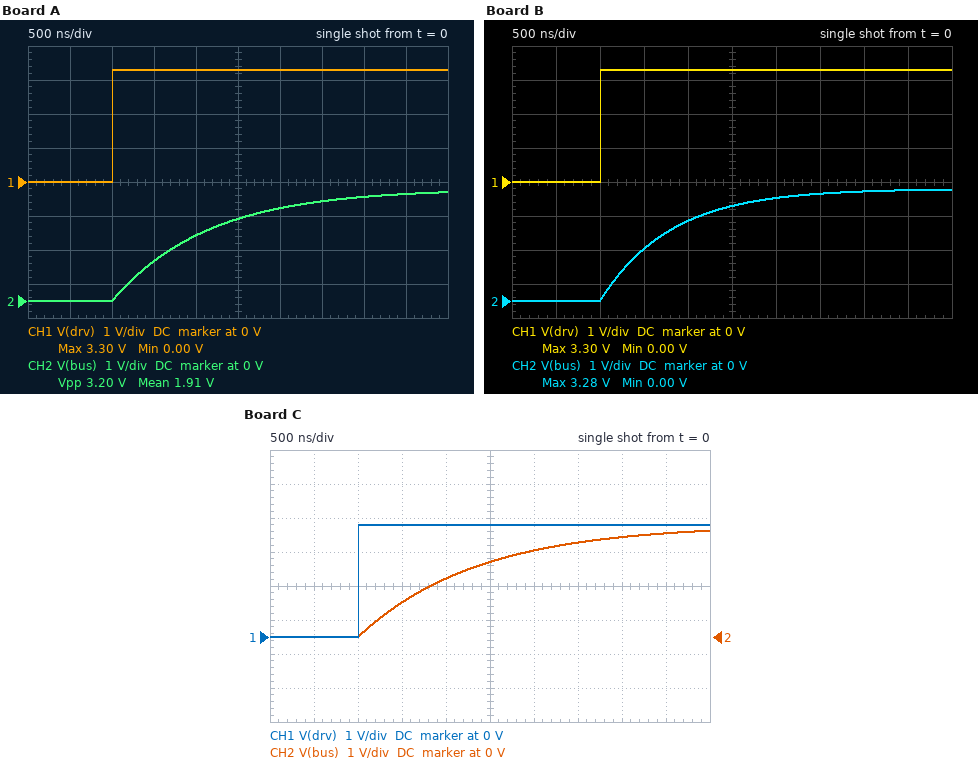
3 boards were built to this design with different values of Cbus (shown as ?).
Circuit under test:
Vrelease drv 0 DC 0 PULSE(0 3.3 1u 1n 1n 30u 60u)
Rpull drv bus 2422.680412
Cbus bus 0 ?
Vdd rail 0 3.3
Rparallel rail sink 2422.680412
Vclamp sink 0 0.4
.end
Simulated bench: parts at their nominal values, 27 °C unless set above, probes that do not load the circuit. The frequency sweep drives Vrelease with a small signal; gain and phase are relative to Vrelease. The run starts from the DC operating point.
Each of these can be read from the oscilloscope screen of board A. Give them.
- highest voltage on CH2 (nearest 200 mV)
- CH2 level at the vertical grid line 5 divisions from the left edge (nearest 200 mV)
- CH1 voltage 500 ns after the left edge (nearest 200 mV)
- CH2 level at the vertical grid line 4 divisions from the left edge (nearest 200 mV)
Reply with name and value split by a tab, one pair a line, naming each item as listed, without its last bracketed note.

highest voltage on CH2	3.2 V
CH2 level at the vertical grid line 5 divisions from the left edge	2.4 V
CH1 voltage 500 ns after the left edge	0 V
CH2 level at the vertical grid line 4 divisions from the left edge	2.0 V
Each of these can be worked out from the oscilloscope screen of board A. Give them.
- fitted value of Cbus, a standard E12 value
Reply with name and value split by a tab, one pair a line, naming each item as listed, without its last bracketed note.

fitted value of Cbus, a standard E12 value	470 pF
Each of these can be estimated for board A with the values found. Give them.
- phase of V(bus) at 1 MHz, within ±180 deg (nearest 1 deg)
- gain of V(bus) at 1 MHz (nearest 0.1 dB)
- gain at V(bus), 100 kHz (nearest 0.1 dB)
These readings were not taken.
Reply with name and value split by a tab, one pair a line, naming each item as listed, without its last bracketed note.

phase of V(bus) at 1 MHz, within ±180 deg	-82 deg
gain of V(bus) at 1 MHz	-17.2 dB
gain at V(bus), 100 kHz	-1.8 dB
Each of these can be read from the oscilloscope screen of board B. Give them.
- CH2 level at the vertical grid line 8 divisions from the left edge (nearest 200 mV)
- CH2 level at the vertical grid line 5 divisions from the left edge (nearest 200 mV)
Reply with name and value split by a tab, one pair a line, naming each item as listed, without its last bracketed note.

CH2 level at the vertical grid line 8 divisions from the left edge	3.2 V
CH2 level at the vertical grid line 5 divisions from the left edge	2.8 V
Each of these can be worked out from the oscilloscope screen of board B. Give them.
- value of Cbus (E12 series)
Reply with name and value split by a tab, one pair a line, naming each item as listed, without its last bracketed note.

value of Cbus	330 pF
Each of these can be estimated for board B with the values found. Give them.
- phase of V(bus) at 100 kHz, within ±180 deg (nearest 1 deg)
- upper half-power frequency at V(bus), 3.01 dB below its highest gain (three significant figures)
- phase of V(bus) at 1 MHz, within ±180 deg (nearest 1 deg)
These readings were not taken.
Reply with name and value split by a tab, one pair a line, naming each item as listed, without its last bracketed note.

phase of V(bus) at 100 kHz, within ±180 deg	-27 deg
upper half-power frequency at V(bus), 3.01 dB below its highest gain	199 kHz
phase of V(bus) at 1 MHz, within ±180 deg	-79 deg
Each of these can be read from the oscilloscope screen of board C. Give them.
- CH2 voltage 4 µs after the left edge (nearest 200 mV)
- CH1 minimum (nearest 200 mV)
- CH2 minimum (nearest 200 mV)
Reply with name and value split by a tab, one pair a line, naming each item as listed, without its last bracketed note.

CH2 voltage 4 µs after the left edge	3.0 V
CH1 minimum	0 V
CH2 minimum	0 V
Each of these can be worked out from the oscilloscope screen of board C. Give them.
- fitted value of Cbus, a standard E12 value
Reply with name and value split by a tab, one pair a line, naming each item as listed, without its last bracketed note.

fitted value of Cbus, a standard E12 value	560 pF
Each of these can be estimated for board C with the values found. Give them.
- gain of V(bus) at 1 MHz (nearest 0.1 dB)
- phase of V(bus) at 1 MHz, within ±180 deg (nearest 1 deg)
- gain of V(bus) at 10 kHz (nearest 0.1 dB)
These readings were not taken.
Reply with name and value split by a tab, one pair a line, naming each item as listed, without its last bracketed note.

gain of V(bus) at 1 MHz	-18.7 dB
phase of V(bus) at 1 MHz, within ±180 deg	-83 deg
gain of V(bus) at 10 kHz	0 dB
